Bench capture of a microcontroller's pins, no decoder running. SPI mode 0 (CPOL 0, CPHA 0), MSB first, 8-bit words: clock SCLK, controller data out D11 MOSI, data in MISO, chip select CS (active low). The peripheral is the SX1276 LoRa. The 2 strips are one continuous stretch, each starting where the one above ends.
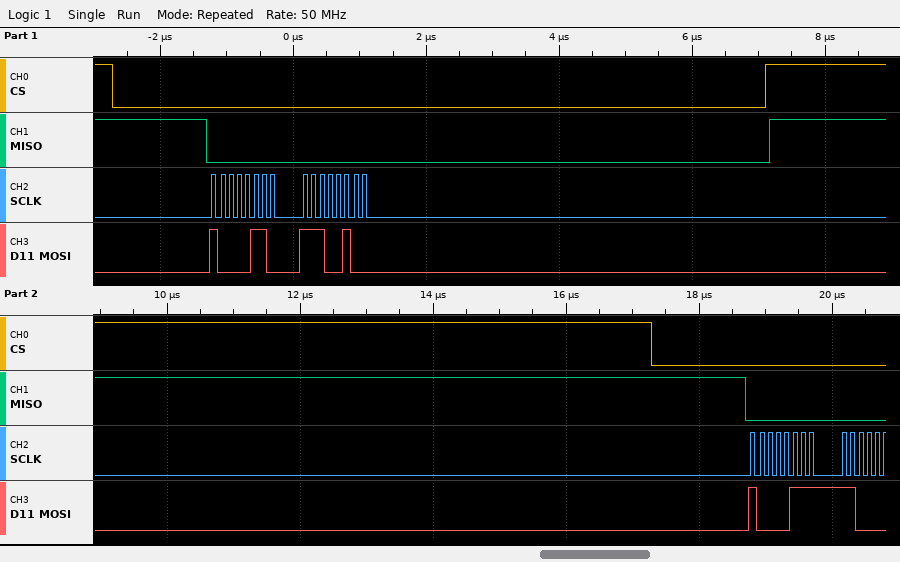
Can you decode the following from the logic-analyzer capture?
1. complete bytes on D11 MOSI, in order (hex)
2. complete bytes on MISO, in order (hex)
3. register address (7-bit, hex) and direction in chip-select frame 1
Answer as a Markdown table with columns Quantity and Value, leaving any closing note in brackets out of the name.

| Quantity | Value |
|---|---|
| complete bytes on D11 MOSI, in order | 86 E4 87 |
| complete bytes on MISO, in order | 00 00 00 |
| register address (7-bit, hex) and direction in chip-select frame 1 | 0x06 write |
